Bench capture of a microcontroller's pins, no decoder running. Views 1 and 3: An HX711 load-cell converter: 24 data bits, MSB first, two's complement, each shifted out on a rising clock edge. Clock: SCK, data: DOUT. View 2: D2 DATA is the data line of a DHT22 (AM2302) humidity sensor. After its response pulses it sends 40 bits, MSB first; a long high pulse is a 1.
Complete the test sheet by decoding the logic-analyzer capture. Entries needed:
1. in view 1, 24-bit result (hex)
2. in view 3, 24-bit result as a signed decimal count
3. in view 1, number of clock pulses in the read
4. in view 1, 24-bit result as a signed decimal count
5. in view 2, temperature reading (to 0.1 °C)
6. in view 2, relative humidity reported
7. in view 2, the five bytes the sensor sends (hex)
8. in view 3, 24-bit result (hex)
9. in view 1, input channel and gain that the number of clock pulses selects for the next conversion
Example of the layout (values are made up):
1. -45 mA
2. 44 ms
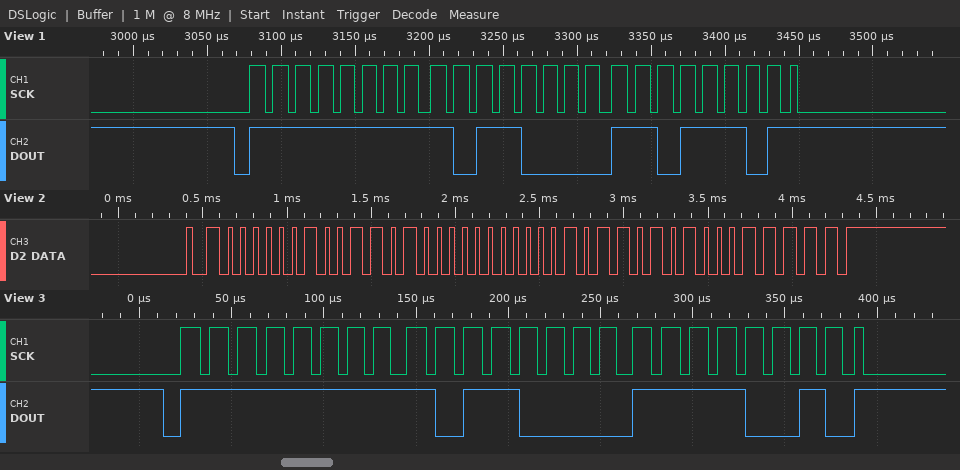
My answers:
1. 0xFFB0DD
2. -20238
3. 25
4. -20259
5. 18.1 °C
6. 61.6 %
7. 02 68 00 B5 1F
8. 0xFFB0F2
9. channel A, gain 128
